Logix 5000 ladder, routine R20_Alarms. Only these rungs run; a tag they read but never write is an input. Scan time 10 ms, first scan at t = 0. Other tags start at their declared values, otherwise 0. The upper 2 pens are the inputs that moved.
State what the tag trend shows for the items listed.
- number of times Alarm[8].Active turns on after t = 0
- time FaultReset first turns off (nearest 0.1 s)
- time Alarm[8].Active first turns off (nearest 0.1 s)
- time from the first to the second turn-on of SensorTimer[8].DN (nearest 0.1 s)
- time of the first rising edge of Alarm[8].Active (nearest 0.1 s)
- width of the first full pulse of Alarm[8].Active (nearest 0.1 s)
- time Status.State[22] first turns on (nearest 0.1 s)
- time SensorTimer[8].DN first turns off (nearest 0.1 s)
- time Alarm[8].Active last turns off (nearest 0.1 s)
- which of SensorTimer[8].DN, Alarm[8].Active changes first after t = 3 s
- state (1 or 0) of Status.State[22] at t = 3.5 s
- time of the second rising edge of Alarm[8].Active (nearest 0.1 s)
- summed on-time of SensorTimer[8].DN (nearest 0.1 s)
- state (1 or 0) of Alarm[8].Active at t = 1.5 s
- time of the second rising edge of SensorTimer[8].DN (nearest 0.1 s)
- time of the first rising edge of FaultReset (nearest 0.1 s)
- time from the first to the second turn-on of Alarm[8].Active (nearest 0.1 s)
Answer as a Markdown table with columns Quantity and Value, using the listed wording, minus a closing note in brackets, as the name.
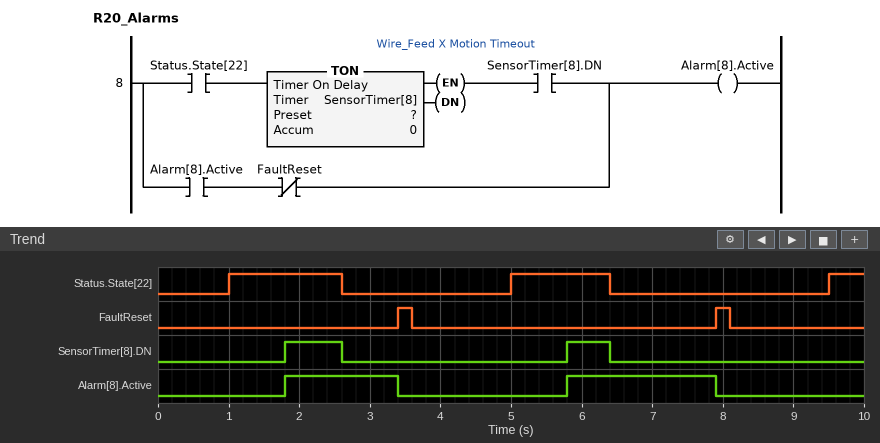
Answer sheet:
| Quantity | Value |
|---|---|
| number of times Alarm[8].Active turns on after t = 0 | 2 |
| time FaultReset first turns off | 3.6 s |
| time Alarm[8].Active first turns off | 3.4 s |
| time from the first to the second turn-on of SensorTimer[8].DN | 4.0 s |
| time of the first rising edge of Alarm[8].Active | 1.8 s |
| width of the first full pulse of Alarm[8].Active | 1.6 s |
| time Status.State[22] first turns on | 1.0 s |
| time SensorTimer[8].DN first turns off | 2.6 s |
| time Alarm[8].Active last turns off | 7.9 s |
| which of SensorTimer[8].DN, Alarm[8].Active changes first after t = 3 s | Alarm[8].Active |
| state (1 or 0) of Status.State[22] at t = 3.5 s | 0 |
| time of the second rising edge of Alarm[8].Active | 5.8 s |
| summed on-time of SensorTimer[8].DN | 1.4 s |
| state (1 or 0) of Alarm[8].Active at t = 1.5 s | 0 |
| time of the second rising edge of SensorTimer[8].DN | 5.8 s |
| time of the first rising edge of FaultReset | 3.4 s |
| time from the first to the second turn-on of Alarm[8].Active | 4.0 s |
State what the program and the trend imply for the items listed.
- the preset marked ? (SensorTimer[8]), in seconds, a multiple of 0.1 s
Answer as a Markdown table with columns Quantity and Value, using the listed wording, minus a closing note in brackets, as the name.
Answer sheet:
| Quantity | Value |
|---|---|
| the preset marked ? (SensorTimer[8]), in seconds, a multiple of 0.1 s | 0.8 s |
